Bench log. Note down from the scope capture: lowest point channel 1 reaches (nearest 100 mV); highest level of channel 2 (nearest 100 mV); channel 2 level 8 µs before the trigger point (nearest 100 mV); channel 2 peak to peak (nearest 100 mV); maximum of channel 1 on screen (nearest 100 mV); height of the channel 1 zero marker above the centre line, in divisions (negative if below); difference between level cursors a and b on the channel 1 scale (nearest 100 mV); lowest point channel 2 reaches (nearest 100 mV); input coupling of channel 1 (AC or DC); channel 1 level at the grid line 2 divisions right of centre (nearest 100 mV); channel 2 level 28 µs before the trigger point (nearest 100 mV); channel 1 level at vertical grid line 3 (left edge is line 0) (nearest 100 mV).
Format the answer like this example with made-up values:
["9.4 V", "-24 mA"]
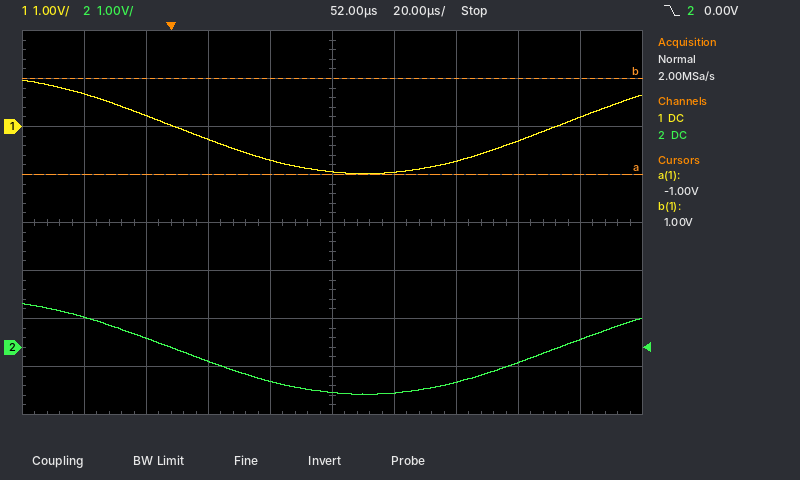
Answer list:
["-1.0 V", "900 mV", "200 mV", "1.9 V", "1.0 V", "+2.0 div", "2.0 V", "-1.0 V", "DC", "-700 mV", "600 mV", "-300 mV"]
